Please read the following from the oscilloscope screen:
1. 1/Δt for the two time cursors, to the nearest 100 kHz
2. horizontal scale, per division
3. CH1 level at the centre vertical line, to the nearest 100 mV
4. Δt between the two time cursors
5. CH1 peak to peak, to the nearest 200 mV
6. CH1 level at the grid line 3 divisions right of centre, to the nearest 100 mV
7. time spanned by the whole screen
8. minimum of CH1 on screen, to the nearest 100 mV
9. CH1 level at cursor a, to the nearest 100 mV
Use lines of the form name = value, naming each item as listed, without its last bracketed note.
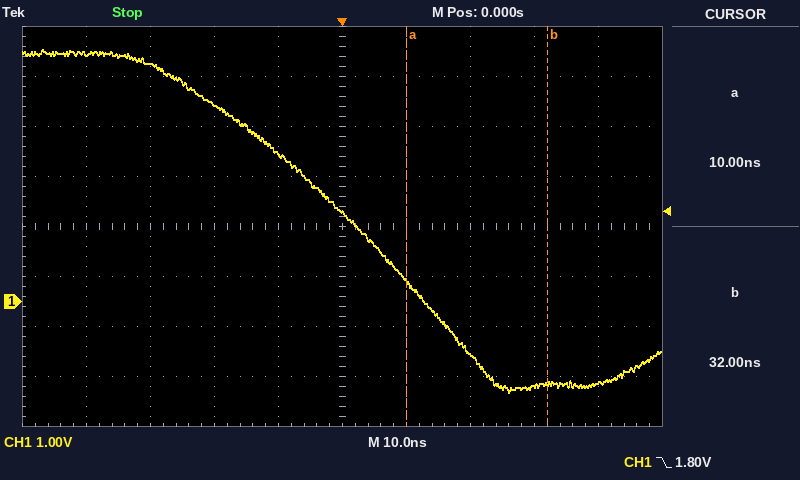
1/Δt for the two time cursors, to the nearest 100 kHz = 45.5 MHz
horizontal scale, per division = 10 ns
CH1 level at the centre vertical line, to the nearest 100 mV = 1.8 V
Δt between the two time cursors = 22 ns
CH1 peak to peak, to the nearest 200 mV = 6.8 V
CH1 level at the grid line 3 divisions right of centre, to the nearest 100 mV = -1.7 V
time spanned by the whole screen = 100 ns
minimum of CH1 on screen, to the nearest 100 mV = -1.8 V
CH1 level at cursor a, to the nearest 100 mV = 400 mV
